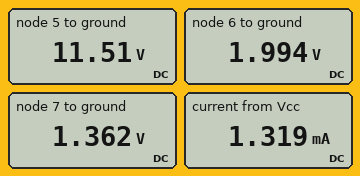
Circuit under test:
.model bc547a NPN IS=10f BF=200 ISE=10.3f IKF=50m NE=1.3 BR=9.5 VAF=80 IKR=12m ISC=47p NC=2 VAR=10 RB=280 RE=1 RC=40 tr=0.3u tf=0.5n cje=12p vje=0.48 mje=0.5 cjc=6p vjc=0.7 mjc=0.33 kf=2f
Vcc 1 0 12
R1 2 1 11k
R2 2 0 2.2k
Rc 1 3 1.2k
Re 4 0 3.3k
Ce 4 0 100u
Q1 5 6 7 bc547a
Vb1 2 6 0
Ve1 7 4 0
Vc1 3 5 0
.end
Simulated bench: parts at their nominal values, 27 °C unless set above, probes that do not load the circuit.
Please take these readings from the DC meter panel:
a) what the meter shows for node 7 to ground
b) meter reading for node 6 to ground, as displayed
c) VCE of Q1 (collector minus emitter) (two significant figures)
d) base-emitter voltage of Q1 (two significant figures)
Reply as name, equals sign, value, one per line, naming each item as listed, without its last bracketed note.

what the meter shows for node 7 to ground = 1.362 V
meter reading for node 6 to ground, as displayed = 1.994 V
VCE of Q1 (collector minus emitter) = 10 V
base-emitter voltage of Q1 = 630 mV
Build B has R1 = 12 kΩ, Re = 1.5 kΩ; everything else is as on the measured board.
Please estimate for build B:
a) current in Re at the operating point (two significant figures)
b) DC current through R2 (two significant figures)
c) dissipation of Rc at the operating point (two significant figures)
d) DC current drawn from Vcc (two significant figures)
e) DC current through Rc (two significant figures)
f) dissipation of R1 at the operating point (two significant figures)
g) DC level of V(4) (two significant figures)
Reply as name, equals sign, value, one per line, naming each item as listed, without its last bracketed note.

current in Re at the operating point = 800 µA
DC current through R2 = 840 µA
dissipation of Rc at the operating point = 750 µW
DC current drawn from Vcc = 1.6 mA
DC current through Rc = 790 µA
dissipation of R1 at the operating point = 8.6 mW
DC level of V(4) = 1.2 V
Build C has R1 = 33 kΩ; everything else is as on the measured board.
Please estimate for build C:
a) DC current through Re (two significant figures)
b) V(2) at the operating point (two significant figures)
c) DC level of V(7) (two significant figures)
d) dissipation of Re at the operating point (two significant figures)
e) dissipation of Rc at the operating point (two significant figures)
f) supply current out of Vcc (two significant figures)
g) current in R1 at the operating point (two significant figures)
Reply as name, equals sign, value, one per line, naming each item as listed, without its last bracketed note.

DC current through Re = 52 µA
V(2) at the operating point = 750 mV
DC level of V(7) = 170 mV
dissipation of Re at the operating point = 9.0 µW
dissipation of Rc at the operating point = 3.2 µW
supply current out of Vcc = 390 µA
current in R1 at the operating point = 340 µA
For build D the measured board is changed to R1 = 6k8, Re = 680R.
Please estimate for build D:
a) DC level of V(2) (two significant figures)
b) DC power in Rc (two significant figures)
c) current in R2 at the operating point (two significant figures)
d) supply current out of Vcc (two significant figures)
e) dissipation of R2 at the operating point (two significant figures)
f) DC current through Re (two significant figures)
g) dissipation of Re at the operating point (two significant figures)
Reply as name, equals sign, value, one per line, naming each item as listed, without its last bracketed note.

DC level of V(2) = 2.9 V
DC power in Rc = 12 mW
current in R2 at the operating point = 1.3 mA
supply current out of Vcc = 4.5 mA
dissipation of R2 at the operating point = 3.8 mW
DC current through Re = 3.2 mA
dissipation of Re at the operating point = 7.1 mW
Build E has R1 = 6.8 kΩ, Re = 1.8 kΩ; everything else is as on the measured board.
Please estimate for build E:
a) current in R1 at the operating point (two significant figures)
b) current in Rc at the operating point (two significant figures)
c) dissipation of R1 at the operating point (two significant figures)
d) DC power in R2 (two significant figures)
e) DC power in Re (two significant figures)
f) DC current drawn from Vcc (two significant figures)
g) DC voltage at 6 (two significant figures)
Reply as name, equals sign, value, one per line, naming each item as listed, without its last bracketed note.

current in R1 at the operating point = 1.3 mA
current in Rc at the operating point = 1.2 mA
dissipation of R1 at the operating point = 12 mW
DC power in R2 = 3.9 mW
DC power in Re = 2.8 mW
DC current drawn from Vcc = 2.6 mA
DC voltage at 6 = 2.9 V
